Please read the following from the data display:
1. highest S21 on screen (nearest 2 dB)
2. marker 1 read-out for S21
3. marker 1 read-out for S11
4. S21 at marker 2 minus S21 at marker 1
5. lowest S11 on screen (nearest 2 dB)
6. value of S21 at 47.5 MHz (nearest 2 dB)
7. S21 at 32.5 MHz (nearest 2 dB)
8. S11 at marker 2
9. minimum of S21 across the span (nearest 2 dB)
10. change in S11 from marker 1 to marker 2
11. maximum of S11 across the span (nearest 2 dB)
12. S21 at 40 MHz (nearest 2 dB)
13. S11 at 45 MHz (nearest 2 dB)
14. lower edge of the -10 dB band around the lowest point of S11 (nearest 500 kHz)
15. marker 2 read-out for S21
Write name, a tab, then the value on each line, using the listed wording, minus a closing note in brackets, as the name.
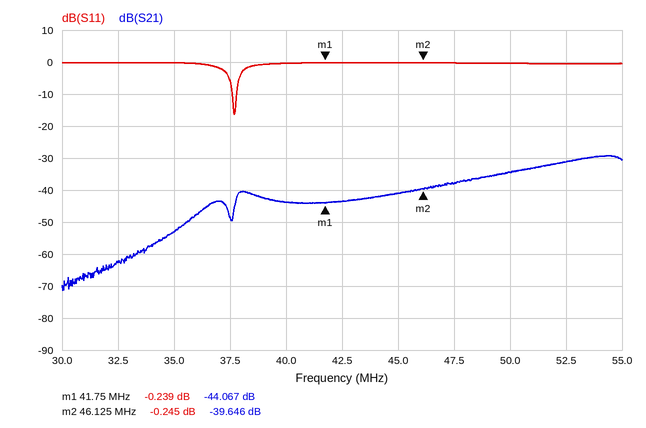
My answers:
highest S21 on screen	-30 dB
marker 1 read-out for S21	-44.067 dB
marker 1 read-out for S11	-0.239 dB
S21 at marker 2 minus S21 at marker 1	4.421 dB
lowest S11 on screen	-16 dB
value of S21 at 47.5 MHz	-38 dB
S21 at 32.5 MHz	-62 dB
S11 at marker 2	-0.245 dB
minimum of S21 across the span	-72 dB
change in S11 from marker 1 to marker 2	-0.006 dB
maximum of S11 across the span	0 dB
S21 at 40 MHz	-44 dB
S11 at 45 MHz	0 dB
lower edge of the -10 dB band around the lowest point of S11	37.5 MHz
marker 2 read-out for S21	-39.646 dB
